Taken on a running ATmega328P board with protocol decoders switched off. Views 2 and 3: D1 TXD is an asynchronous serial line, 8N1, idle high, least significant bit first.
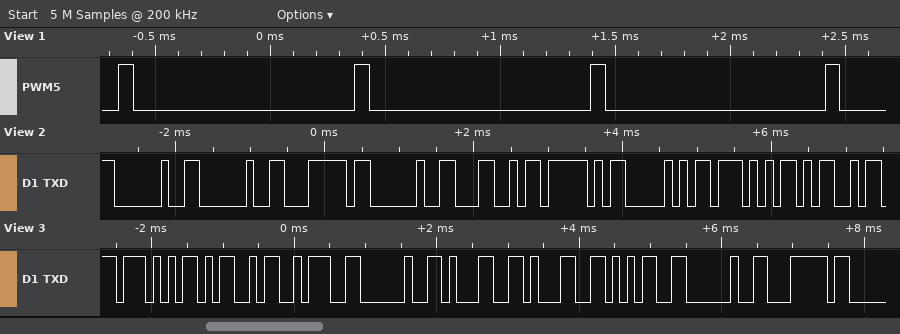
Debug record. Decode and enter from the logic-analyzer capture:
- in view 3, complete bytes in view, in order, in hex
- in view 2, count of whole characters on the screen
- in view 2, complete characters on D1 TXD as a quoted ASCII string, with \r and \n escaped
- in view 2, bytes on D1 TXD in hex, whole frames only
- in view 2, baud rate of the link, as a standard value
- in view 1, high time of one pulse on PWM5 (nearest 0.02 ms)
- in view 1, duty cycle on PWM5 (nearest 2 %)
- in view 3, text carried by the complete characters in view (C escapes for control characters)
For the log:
57 4D 3A 20 31 31 35 20 7C
9
"  | L_PWM"
20 20 7C 20 4C 5F 50 57 4D
9600 baud
0.06 ms
6 %
"WM: 115 |"
